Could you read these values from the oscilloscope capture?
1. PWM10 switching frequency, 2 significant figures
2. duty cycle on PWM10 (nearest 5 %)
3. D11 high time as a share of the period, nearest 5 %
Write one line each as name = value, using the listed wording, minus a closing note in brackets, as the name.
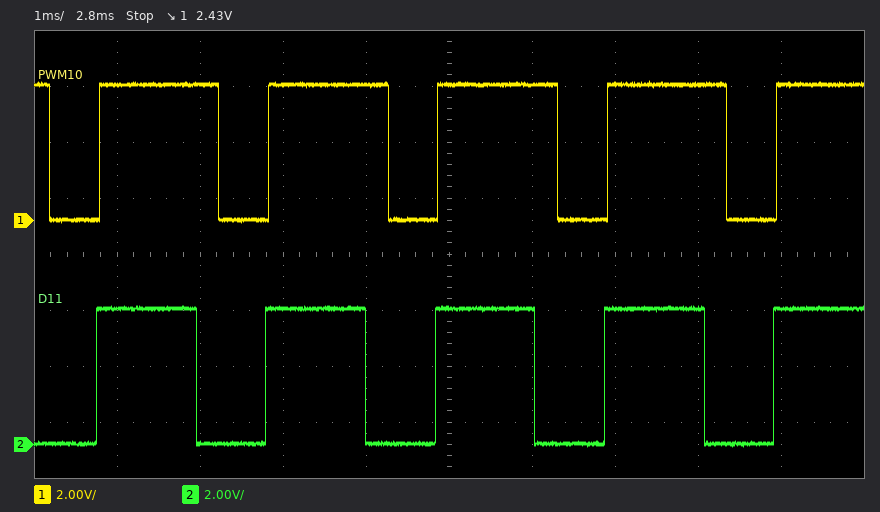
PWM10 switching frequency, 2 significant figures = 490 Hz
duty cycle on PWM10 = 70 %
D11 high time as a share of the period, nearest 5 % = 60 %
